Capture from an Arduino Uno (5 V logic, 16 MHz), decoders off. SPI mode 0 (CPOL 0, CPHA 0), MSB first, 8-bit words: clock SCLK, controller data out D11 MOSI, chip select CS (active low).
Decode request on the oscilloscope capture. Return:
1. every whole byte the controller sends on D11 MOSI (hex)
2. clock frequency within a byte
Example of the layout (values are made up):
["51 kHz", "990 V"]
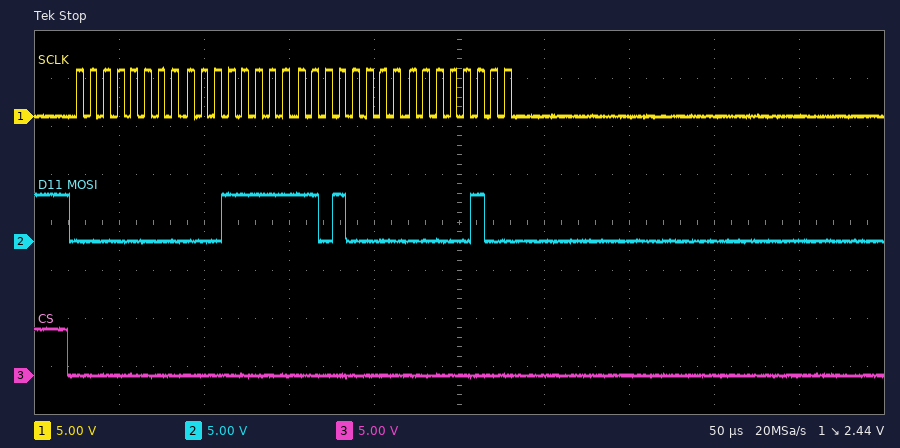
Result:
["00 1F D0 04", "125 kHz"]
